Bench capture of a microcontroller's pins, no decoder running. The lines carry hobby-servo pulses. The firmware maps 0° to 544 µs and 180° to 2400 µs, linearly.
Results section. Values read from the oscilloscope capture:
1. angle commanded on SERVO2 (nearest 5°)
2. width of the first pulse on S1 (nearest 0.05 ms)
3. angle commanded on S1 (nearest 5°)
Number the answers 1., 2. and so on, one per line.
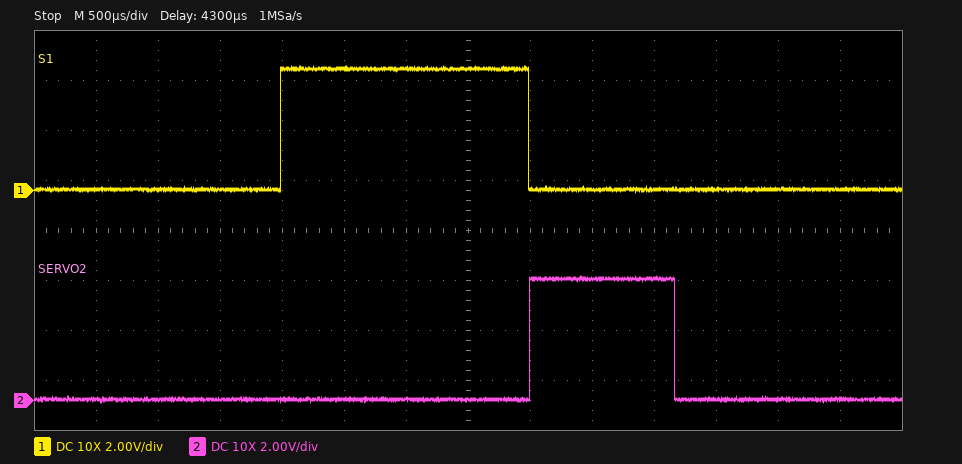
1. 60°
2. 2.00 ms
3. 140°
